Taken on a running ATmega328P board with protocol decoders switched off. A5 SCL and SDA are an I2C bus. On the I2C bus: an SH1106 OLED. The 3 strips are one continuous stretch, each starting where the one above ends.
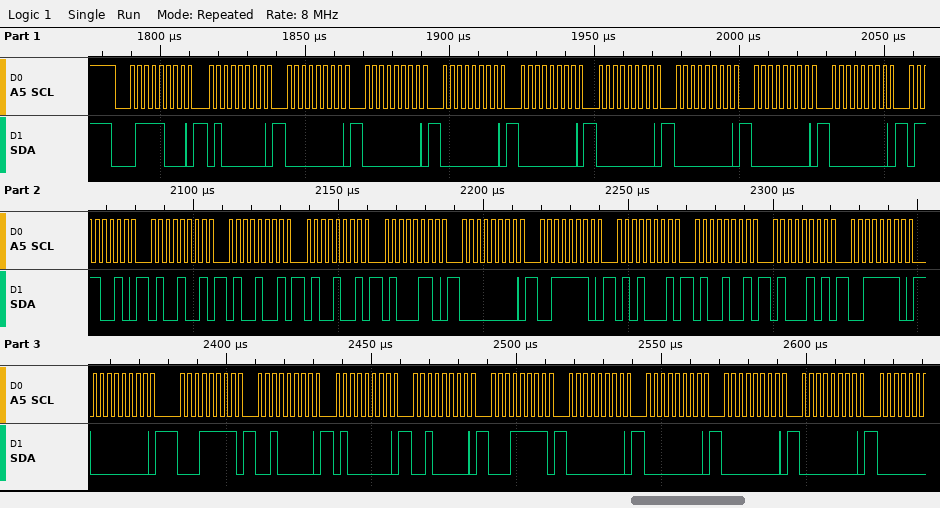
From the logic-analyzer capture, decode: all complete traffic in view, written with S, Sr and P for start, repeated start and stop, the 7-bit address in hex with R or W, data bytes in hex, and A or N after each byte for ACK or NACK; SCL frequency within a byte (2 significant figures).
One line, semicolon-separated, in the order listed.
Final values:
S 3CW A 40 A 00 A 00 A 00 A 00 A 00 A 00 A 00 A 00 A 72 A 49 A 49 A 49 A 46 A 00 A 3E A 51 A 49 A 45 A 3E A 00 A 1F A 20 A 40 A 20 A 1F A 00 A 00 A 00 A 00 A; 400 kHz
